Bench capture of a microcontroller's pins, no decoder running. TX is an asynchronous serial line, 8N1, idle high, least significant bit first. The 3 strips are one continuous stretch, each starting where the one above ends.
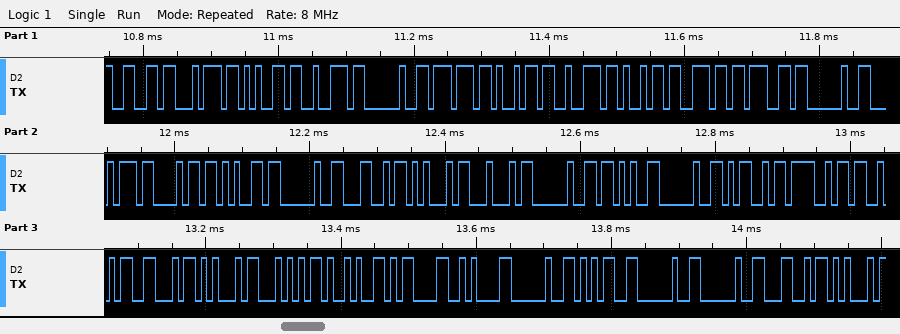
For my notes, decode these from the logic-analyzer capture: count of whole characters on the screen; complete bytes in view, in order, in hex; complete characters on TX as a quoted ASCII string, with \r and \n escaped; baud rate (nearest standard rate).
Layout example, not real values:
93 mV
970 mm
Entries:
37
66 74 65 72 20 77 69 72 69 6E 67 20 74 68 65 20 4C 45 44 20 2B 20 4D 4F 53 46 45 54 29 0D 0A 20 35 20 20 4C 45
"fter wiring the LED + MOSFET)\r\n 5  LE"
115200 baud
